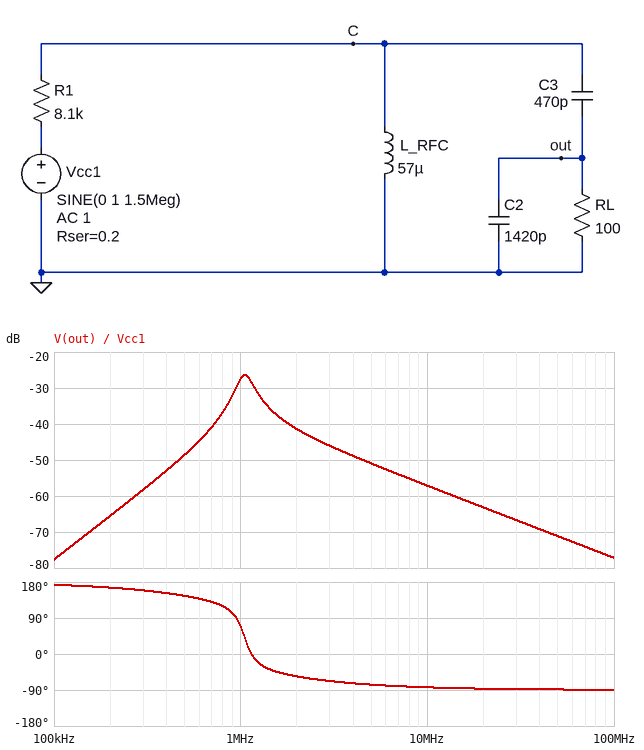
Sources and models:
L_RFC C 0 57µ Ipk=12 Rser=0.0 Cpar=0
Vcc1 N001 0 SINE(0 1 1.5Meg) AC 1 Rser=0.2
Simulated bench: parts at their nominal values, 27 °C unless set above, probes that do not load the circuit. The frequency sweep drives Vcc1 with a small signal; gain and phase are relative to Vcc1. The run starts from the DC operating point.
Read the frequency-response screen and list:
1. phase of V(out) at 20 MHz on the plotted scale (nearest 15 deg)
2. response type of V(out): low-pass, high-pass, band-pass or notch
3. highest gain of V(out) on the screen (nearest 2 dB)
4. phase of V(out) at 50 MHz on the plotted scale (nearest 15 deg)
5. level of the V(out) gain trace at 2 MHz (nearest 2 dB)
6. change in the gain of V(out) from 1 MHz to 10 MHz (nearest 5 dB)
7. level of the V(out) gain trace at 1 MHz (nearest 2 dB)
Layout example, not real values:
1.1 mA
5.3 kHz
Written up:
-90 deg
band-pass
-26 dB
-90 deg
-42 dB
-30 dB
-28 dB
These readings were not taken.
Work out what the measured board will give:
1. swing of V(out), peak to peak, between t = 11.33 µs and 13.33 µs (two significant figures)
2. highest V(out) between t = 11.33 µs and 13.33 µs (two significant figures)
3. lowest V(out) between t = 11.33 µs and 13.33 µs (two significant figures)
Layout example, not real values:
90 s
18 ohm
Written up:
29 mV
15 mV
-15 mV
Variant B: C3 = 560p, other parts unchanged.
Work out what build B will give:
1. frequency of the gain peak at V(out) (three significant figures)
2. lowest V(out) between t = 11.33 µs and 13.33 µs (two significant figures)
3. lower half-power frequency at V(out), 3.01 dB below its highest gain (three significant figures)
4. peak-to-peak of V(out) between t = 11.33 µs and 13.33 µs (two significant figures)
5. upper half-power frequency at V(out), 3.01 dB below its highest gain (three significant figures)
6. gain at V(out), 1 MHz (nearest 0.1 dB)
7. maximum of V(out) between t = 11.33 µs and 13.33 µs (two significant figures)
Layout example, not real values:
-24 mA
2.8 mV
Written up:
974 kHz
-13 mV
875 kHz
26 mV
1.10 MHz
-27.2 dB
13 mV
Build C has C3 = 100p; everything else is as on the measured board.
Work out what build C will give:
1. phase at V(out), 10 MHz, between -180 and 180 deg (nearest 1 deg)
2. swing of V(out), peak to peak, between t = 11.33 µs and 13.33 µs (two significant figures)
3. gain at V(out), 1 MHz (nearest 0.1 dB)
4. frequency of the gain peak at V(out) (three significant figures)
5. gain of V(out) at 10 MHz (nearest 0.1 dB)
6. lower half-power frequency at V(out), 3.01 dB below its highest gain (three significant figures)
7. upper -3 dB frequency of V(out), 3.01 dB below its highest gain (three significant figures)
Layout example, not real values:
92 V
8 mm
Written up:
-82 deg
14 mV
-51.8 dB
2.17 MHz
-56.8 dB
2.04 MHz
2.31 MHz
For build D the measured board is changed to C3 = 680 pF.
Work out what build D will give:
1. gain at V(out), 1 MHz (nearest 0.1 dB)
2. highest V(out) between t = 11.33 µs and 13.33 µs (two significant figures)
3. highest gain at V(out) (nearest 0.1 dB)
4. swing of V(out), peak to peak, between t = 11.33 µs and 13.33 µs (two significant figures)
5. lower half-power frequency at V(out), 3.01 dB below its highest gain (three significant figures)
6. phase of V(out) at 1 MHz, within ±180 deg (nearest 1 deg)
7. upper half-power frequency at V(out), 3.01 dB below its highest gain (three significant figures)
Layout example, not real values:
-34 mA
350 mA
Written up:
-29.9 dB
12 mV
-27.6 dB
23 mV
791 kHz
0 deg
1.03 MHz
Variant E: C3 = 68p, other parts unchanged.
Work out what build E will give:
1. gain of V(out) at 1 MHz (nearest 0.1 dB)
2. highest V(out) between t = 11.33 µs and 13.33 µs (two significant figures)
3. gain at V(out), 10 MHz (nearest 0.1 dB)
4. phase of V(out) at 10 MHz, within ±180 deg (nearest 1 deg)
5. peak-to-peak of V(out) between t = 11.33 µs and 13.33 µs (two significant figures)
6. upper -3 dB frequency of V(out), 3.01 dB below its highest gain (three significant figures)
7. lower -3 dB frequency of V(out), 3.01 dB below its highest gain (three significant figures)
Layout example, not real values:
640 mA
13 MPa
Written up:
-55.8 dB
3.7 mV
-56.6 dB
-82 deg
7.4 mV
2.79 MHz
2.44 MHz
